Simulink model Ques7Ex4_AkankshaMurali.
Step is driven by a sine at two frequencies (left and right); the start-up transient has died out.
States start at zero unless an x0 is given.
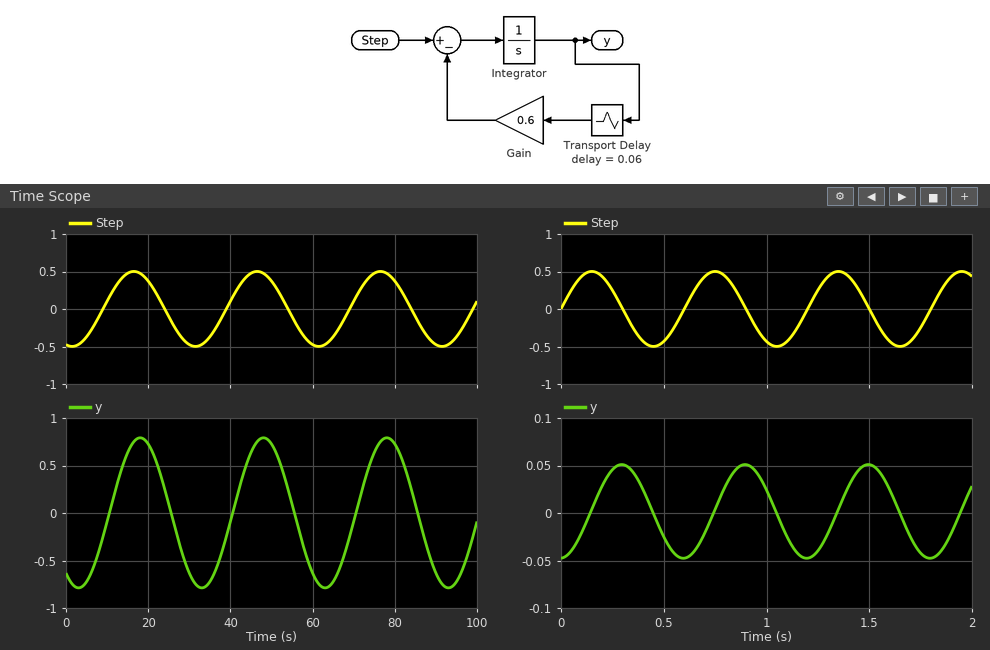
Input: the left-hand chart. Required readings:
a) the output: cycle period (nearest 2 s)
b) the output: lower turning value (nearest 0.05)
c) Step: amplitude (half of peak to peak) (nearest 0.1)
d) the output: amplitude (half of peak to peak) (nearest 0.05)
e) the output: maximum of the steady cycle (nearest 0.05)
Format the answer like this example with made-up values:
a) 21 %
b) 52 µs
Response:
a) 30 s
b) -0.80
c) 0.5
d) 0.80
e) 0.80
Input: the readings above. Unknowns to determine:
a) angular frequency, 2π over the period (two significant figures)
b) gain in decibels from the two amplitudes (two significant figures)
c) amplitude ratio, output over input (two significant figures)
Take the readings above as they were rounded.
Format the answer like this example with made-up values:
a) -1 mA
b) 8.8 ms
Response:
a) 0.21 rad/s
b) 4.1 dB
c) 1.6
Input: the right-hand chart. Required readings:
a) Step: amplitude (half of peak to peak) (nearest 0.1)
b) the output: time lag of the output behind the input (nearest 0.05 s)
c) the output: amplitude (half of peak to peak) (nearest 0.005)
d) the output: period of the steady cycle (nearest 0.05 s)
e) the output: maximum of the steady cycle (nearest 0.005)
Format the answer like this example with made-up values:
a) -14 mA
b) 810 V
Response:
a) 0.5
b) 0.15 s
c) 0.050
d) 0.60 s
e) 0.050
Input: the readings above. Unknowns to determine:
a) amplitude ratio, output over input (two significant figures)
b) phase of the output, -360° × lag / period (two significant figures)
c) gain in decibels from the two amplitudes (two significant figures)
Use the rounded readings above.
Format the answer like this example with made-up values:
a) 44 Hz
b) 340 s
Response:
a) 0.10
b) -90°
c) -20 dB
